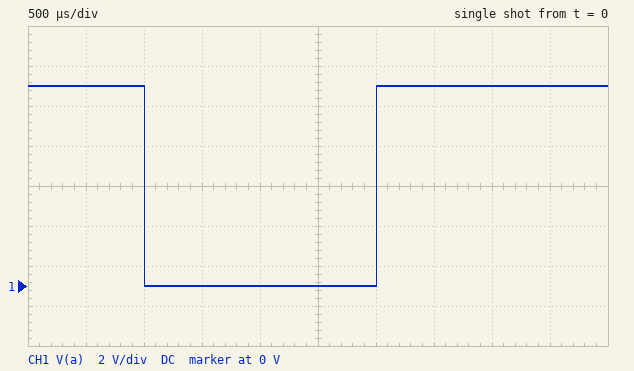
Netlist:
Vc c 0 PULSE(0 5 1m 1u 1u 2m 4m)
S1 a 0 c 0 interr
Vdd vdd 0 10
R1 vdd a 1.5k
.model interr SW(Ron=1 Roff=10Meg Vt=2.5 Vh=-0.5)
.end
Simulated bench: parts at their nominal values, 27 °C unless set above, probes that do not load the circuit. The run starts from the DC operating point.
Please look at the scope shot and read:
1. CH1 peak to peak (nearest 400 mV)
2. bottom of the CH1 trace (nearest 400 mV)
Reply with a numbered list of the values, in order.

1. 10.0 V
2. 0 V
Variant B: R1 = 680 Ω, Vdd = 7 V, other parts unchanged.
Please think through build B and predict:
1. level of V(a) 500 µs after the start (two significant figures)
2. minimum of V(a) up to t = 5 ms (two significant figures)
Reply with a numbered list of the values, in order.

1. 7.0 V
2. 10 mV
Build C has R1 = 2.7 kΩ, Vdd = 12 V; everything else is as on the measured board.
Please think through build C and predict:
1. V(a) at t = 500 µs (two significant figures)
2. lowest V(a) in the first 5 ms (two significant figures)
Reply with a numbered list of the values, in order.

1. 12 V
2. 4.4 mV
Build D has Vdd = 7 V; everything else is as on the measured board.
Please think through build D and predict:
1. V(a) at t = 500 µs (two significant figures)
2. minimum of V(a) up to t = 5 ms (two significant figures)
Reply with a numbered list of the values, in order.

1. 7.0 V
2. 4.7 mV
